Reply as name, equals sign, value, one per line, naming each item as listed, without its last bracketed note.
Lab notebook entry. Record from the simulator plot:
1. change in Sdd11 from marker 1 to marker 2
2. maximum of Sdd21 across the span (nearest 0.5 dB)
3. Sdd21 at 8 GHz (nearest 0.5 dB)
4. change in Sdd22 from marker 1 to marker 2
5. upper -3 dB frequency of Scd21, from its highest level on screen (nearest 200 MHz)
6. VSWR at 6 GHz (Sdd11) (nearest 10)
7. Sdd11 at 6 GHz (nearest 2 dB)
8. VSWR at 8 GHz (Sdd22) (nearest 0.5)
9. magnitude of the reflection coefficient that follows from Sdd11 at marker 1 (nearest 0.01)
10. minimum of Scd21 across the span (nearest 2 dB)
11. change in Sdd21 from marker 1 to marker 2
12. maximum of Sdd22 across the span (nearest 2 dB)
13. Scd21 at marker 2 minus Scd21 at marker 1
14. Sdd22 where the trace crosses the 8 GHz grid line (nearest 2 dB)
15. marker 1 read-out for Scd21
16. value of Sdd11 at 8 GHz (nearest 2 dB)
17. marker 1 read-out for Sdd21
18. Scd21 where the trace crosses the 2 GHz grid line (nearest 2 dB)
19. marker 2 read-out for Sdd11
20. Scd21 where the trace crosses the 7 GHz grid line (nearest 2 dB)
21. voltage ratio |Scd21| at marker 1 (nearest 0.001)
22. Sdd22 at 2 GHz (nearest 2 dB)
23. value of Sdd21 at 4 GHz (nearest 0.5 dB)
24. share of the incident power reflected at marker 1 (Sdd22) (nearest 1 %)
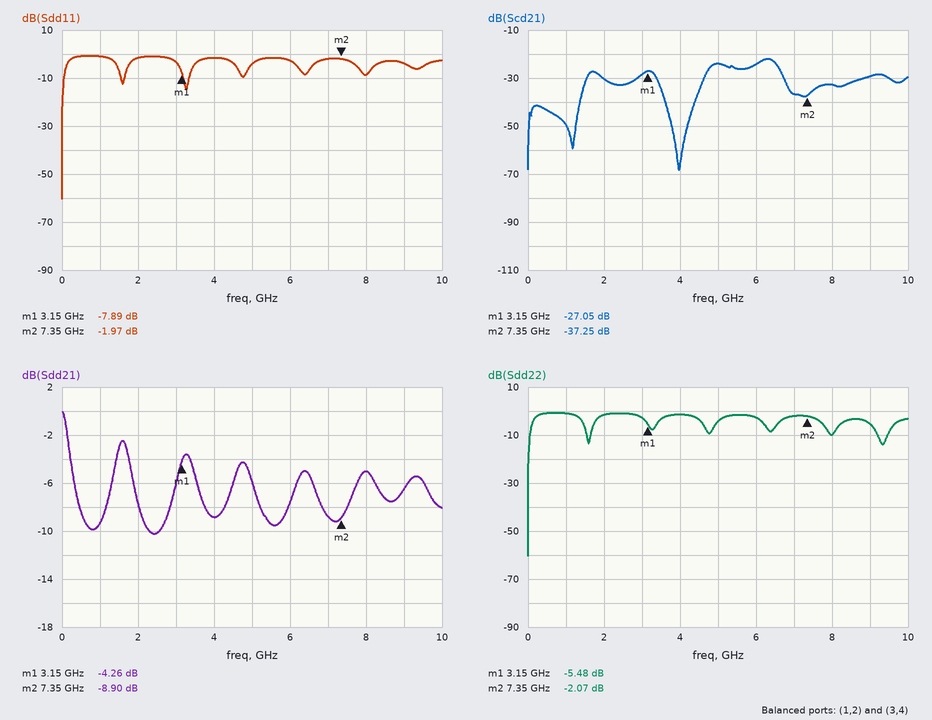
change in Sdd11 from marker 1 to marker 2 = 5.92 dB
maximum of Sdd21 across the span = 0.0 dB
Sdd21 at 8 GHz = -5.0 dB
change in Sdd22 from marker 1 to marker 2 = 3.41 dB
upper -3 dB frequency of Scd21, from its highest level on screen = 6.6 GHz
VSWR at 6 GHz (Sdd11) = 10
Sdd11 at 6 GHz = -2 dB
VSWR at 8 GHz (Sdd22) = 2.0
magnitude of the reflection coefficient that follows from Sdd11 at marker 1 = 0.40
minimum of Scd21 across the span = -68 dB
change in Sdd21 from marker 1 to marker 2 = -4.64 dB
maximum of Sdd22 across the span = 0 dB
Scd21 at marker 2 minus Scd21 at marker 1 = -10.20 dB
Sdd22 where the trace crosses the 8 GHz grid line = -10 dB
marker 1 read-out for Scd21 = -27.05 dB
value of Sdd11 at 8 GHz = -8 dB
marker 1 read-out for Sdd21 = -4.26 dB
Scd21 where the trace crosses the 2 GHz grid line = -30 dB
marker 2 read-out for Sdd11 = -1.97 dB
Scd21 where the trace crosses the 7 GHz grid line = -36 dB
voltage ratio |Scd21| at marker 1 = 0.044
Sdd22 at 2 GHz = -2 dB
value of Sdd21 at 4 GHz = -9.0 dB
share of the incident power reflected at marker 1 (Sdd22) = 28 %
